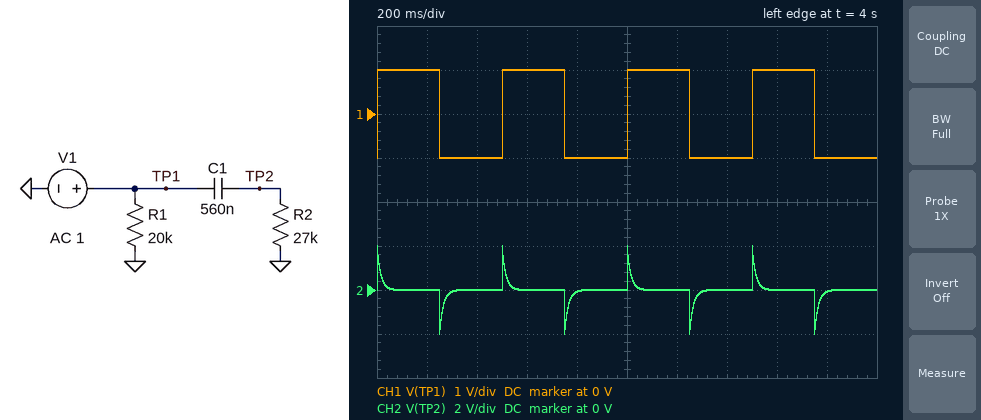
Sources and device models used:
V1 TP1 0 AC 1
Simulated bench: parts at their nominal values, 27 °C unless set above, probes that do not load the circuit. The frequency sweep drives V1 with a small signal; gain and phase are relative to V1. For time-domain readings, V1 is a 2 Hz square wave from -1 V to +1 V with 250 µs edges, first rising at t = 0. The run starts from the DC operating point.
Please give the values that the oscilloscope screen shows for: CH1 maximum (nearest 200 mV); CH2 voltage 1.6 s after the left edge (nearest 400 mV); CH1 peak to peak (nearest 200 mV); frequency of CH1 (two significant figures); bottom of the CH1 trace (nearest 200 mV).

1.0 V
0 V
2.0 V
2.0 Hz
-1.0 V
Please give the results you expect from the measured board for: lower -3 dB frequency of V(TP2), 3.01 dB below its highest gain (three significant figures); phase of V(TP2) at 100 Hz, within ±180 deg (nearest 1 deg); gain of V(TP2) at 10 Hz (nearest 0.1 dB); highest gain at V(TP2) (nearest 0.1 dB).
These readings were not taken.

10.5 Hz
6 deg
-3.2 dB
0 dB
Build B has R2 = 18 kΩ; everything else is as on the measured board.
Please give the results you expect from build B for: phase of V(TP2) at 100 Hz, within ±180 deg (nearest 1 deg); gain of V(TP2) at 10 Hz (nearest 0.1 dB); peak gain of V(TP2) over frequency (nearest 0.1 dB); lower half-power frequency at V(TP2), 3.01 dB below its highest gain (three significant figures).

9 deg
-5.4 dB
0 dB
15.8 Hz
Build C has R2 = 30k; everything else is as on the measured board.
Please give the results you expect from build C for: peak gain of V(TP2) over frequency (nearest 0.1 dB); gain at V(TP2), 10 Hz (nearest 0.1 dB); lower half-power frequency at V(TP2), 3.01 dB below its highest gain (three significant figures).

0 dB
-2.8 dB
9.47 Hz
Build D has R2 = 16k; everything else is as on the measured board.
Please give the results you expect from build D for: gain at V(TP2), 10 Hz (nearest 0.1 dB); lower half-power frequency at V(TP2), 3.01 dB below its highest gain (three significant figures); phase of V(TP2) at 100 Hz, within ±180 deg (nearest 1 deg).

-6.2 dB
17.8 Hz
10 deg
